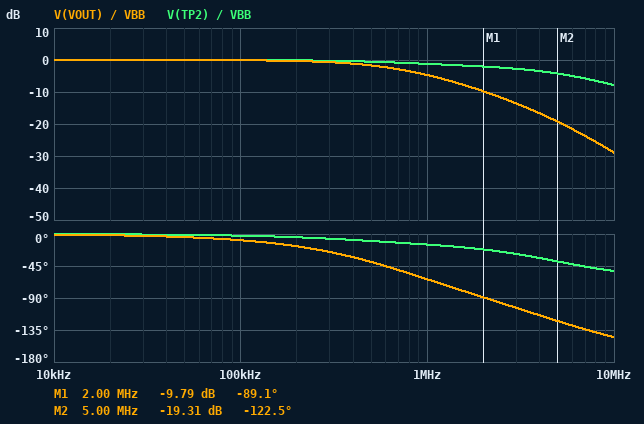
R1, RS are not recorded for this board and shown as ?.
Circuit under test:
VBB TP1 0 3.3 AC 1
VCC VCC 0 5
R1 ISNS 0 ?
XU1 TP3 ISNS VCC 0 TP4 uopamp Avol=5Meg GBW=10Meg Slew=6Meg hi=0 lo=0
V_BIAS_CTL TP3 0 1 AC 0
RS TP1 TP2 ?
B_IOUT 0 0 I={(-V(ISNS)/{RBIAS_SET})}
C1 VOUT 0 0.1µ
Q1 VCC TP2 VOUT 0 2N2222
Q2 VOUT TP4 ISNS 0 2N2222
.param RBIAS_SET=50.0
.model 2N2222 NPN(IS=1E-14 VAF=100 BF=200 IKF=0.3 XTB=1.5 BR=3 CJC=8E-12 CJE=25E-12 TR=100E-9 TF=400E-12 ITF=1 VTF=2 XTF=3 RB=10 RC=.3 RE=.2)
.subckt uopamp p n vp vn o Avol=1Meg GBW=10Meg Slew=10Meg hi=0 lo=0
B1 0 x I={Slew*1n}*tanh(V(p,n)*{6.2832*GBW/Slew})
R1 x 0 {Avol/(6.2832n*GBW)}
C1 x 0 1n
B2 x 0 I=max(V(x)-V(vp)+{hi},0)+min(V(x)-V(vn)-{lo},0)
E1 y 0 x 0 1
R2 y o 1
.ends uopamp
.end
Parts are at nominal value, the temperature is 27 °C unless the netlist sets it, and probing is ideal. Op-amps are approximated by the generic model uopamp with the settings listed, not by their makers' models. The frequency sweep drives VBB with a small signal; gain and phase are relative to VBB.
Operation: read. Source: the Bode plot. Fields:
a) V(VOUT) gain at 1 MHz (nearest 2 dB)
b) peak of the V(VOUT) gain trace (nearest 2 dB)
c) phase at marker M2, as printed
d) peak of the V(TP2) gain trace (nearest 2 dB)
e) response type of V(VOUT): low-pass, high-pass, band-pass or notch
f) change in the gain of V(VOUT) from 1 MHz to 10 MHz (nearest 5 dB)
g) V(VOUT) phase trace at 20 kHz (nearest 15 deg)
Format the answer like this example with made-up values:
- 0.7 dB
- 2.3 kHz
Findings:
- -4 dB
- 0 dB
- -122.5 deg
- 0 dB
- low-pass
- -25 dB
- 0 deg
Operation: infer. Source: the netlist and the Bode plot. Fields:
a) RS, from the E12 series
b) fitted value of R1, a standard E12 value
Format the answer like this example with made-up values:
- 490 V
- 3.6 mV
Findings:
- 120 Ω
- 56 Ω
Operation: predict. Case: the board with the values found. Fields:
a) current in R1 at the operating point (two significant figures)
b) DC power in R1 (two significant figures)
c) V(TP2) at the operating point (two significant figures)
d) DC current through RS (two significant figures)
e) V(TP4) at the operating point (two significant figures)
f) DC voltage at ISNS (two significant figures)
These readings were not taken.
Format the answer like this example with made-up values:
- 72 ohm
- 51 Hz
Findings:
- 18 mA
- 18 mW
- 3.3 V
- 92 µA
- 1.7 V
- 1.0 V
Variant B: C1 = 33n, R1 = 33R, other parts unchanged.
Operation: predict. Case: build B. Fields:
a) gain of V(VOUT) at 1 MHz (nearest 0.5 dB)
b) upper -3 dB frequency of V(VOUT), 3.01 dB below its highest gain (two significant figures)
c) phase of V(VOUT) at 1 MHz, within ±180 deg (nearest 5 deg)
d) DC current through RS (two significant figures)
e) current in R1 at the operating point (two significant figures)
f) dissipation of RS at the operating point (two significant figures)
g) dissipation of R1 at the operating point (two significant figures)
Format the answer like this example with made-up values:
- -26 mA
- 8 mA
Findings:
- 0 dB
- 3.5 MHz
- -25 deg
- 160 µA
- 30 mA
- 3.1 µW
- 30 mW
